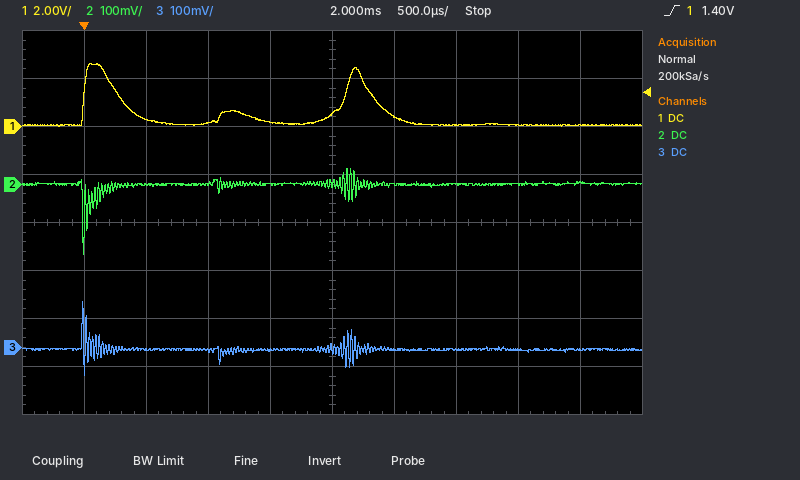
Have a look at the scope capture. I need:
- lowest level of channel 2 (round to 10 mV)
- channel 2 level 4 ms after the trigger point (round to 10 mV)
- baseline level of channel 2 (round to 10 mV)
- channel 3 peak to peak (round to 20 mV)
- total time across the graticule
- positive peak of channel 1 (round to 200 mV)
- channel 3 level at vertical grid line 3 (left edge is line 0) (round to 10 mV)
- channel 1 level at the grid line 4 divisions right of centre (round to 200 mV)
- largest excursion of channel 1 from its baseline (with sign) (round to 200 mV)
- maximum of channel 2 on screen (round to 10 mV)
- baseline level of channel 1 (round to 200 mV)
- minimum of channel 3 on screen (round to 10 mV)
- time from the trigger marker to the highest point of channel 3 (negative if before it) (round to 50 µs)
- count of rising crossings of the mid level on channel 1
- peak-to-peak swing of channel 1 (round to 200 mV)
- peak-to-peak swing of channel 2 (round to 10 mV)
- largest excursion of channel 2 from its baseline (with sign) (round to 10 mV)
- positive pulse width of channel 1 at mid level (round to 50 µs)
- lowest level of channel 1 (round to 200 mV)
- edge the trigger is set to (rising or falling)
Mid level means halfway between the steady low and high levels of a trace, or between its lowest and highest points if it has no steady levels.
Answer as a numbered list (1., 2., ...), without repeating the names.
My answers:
1. -150 mV
2. 0 mV
3. 0 mV
4. 160 mV
5. 5 ms
6. 2.6 V
7. -10 mV
8. 0.0 V
9. +2.6 V
10. 30 mV
11. 0.0 V
12. -60 mV
13. 0 µs
14. 2
15. 2.6 V
16. 180 mV
17. -150 mV
18. 250 µs
19. 0.0 V
20. rising
